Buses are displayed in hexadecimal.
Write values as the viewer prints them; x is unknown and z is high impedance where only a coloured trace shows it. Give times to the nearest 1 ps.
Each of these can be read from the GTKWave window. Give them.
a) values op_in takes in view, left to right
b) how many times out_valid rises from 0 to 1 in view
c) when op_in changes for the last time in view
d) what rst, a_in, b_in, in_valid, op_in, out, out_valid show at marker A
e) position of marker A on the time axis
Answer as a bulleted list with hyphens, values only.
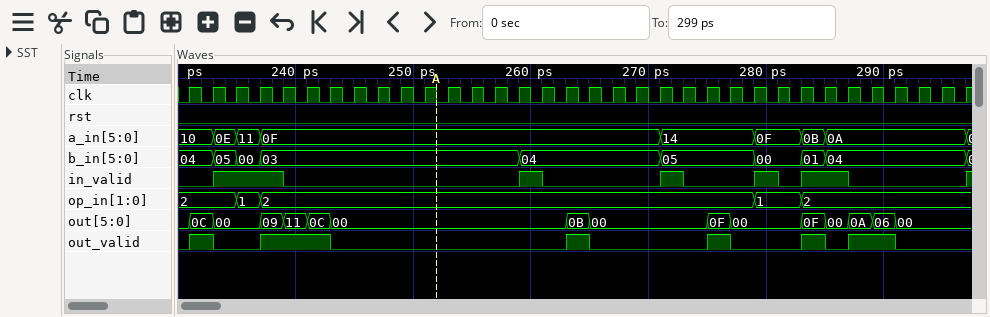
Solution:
- 2, 1, 2, 1, 2
- 6
- 283 ps
- rst=0, a_in=0F, b_in=03, in_valid=0, op_in=2, out=00, out_valid=0
- 252 ps
